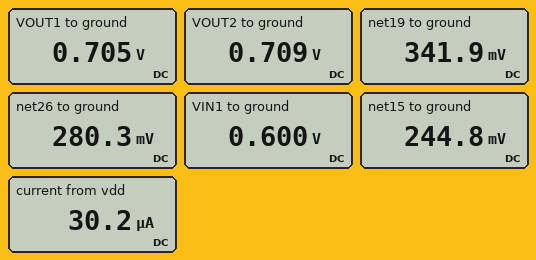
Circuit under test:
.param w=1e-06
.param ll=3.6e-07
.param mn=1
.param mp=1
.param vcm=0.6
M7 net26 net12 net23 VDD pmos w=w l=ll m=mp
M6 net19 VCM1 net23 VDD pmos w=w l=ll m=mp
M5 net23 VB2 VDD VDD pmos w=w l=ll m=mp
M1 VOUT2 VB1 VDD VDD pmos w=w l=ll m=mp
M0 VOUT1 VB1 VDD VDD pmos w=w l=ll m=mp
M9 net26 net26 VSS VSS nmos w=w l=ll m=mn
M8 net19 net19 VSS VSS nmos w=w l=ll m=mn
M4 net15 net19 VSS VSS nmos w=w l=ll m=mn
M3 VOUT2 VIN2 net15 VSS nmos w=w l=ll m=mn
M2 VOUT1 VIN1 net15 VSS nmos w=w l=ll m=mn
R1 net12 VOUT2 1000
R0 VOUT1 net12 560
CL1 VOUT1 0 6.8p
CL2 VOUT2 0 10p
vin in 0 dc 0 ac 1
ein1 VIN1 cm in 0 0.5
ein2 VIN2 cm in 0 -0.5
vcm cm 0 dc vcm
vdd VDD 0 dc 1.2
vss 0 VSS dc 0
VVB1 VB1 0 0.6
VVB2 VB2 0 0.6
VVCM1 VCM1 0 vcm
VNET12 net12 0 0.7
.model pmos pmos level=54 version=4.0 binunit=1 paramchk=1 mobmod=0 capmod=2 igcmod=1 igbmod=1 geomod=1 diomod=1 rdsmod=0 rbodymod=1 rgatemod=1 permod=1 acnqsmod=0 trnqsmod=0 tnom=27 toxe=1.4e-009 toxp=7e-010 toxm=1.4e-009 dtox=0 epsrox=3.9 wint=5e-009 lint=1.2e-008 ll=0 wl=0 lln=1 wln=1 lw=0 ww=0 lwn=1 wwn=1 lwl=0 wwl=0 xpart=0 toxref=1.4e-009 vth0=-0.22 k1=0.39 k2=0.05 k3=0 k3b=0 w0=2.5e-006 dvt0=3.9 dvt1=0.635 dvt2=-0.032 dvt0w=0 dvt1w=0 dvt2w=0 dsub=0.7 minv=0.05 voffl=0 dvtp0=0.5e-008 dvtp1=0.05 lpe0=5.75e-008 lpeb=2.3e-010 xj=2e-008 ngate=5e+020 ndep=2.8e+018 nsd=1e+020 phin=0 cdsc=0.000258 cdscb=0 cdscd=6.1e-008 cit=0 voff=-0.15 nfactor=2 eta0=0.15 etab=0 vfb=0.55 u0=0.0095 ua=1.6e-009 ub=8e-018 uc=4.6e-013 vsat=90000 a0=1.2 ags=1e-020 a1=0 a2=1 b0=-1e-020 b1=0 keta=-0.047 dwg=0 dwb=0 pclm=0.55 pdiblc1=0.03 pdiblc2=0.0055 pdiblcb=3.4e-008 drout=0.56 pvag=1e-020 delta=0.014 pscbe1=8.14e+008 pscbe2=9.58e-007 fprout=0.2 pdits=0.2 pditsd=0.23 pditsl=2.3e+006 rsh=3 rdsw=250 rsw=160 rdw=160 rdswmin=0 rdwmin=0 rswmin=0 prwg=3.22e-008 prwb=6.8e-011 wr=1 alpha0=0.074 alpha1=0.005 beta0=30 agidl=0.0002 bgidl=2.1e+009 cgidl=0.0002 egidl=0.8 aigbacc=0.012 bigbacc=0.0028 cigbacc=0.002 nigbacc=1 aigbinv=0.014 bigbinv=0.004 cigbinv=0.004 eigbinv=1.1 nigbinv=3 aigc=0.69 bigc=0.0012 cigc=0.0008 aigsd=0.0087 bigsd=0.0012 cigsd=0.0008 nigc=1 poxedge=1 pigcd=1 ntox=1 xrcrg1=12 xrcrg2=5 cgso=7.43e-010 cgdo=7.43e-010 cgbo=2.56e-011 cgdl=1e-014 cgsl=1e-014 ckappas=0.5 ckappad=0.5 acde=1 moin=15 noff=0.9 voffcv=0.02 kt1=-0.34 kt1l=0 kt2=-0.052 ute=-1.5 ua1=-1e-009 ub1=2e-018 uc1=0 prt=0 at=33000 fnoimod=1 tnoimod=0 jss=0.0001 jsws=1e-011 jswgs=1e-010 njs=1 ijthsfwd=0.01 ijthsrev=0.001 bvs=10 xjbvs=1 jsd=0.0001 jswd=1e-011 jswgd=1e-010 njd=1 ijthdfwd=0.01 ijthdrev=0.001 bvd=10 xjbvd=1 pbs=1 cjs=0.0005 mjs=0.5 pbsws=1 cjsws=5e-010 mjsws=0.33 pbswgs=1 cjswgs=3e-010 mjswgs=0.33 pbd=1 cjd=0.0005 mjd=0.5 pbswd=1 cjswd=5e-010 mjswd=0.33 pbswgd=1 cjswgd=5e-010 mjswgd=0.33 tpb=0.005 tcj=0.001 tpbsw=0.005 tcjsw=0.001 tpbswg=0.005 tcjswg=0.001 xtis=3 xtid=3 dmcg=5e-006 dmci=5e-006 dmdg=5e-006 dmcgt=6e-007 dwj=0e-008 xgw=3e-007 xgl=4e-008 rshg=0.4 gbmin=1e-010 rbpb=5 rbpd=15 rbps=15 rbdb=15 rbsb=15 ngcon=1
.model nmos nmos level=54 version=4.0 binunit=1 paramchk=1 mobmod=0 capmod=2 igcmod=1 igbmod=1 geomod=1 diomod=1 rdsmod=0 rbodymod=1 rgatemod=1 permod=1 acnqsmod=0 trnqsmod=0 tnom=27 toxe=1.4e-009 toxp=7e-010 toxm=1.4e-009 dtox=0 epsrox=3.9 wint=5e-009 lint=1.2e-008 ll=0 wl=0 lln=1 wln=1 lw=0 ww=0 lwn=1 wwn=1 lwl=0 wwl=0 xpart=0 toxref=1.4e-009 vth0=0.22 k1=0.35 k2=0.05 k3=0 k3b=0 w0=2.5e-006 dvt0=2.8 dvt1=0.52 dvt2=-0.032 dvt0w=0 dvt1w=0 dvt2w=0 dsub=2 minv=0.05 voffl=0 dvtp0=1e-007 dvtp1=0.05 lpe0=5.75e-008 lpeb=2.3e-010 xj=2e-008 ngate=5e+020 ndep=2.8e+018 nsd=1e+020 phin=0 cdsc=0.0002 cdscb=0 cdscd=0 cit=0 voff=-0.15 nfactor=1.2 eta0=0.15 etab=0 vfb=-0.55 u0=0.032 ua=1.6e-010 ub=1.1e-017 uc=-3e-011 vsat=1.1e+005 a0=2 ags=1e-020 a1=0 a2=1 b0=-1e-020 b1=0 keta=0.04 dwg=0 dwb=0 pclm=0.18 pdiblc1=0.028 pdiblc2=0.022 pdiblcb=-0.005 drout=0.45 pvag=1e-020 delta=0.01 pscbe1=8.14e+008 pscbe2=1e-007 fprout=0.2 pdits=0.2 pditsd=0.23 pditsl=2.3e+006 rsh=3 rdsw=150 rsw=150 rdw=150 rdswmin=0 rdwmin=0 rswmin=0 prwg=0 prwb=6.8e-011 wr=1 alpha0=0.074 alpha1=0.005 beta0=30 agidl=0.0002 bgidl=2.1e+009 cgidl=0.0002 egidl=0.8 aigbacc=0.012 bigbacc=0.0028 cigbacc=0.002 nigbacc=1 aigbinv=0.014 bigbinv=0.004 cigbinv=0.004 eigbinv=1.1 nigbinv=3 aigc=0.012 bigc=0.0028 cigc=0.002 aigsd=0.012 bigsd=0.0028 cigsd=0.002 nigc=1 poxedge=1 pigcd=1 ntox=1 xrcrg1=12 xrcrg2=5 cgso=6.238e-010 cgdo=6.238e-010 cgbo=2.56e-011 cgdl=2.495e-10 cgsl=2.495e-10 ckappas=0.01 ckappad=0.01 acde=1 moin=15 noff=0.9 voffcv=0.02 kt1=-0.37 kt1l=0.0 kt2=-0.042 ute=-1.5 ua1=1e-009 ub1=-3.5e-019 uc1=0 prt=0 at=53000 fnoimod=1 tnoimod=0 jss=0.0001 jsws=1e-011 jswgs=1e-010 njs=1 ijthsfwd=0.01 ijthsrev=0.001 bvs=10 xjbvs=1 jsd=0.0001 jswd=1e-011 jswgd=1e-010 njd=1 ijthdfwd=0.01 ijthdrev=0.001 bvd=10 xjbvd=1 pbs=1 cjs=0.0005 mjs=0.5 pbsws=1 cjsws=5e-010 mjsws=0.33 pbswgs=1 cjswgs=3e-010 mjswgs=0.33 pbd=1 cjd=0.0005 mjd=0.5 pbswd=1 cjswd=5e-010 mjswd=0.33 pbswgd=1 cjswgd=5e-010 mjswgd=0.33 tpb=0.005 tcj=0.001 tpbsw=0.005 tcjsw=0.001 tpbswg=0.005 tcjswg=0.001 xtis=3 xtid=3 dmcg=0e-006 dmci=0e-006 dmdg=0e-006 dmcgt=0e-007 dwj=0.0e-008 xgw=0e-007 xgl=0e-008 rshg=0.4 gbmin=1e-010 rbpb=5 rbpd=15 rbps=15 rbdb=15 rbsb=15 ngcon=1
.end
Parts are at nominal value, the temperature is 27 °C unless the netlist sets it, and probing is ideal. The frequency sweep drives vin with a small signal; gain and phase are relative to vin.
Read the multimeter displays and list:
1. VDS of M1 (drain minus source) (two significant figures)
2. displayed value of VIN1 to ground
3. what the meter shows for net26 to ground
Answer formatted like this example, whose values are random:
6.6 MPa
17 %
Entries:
-490 mV
0.600 V
280.3 mV
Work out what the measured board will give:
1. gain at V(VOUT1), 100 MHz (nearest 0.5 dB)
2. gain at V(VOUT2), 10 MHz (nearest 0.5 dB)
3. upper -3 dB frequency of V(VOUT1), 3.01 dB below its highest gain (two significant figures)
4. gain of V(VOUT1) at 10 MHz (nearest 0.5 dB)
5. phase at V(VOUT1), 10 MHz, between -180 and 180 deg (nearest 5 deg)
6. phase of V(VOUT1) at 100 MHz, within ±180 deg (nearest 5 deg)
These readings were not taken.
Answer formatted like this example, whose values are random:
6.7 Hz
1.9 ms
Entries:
-48.5 dB
-36.5 dB
42 MHz
-40.5 dB
165 deg
110 deg
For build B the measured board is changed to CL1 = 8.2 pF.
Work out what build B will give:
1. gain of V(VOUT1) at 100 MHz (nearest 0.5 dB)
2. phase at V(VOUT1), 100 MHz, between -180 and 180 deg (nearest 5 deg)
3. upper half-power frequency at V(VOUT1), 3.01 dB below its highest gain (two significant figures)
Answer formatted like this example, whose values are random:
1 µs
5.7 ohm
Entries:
-50.0 dB
105 deg
35 MHz
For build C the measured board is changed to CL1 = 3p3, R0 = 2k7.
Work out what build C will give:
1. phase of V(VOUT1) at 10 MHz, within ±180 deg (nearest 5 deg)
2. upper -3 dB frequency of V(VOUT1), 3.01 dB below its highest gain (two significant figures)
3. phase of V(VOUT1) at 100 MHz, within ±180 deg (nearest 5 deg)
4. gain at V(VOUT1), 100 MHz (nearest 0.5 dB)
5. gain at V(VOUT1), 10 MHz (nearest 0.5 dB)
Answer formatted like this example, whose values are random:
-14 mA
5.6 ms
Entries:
150 deg
18 MHz
100 deg
-41.5 dB
-28.0 dB
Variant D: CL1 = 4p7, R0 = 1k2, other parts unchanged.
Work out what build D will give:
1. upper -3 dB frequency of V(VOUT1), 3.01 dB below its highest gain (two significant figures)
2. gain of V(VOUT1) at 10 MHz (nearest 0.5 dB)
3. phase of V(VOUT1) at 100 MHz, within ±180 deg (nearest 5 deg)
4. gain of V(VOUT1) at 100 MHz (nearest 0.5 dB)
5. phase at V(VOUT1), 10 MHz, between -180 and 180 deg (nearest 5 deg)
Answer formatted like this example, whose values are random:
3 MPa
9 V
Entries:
28 MHz
-34.0 dB
105 deg
-45.0 dB
160 deg
